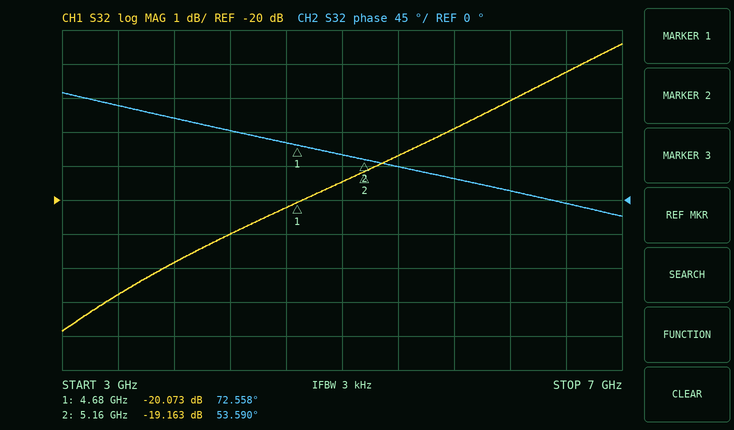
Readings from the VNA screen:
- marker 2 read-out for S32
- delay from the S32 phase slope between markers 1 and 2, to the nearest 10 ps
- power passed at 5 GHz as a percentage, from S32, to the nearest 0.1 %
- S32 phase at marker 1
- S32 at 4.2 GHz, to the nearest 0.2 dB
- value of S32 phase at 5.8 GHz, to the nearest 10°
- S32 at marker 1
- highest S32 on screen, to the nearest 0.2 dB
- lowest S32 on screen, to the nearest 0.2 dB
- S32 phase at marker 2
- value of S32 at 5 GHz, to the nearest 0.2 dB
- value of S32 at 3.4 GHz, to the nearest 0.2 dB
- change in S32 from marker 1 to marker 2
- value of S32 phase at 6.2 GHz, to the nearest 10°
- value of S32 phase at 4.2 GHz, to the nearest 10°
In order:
-19.163 dB
110 ps
1.1 %
72.558°
-21.0 dB
30°
-20.073 dB
-15.4 dB
-23.8 dB
53.590°
-19.4 dB
-22.8 dB
0.910 dB
10°
90°
